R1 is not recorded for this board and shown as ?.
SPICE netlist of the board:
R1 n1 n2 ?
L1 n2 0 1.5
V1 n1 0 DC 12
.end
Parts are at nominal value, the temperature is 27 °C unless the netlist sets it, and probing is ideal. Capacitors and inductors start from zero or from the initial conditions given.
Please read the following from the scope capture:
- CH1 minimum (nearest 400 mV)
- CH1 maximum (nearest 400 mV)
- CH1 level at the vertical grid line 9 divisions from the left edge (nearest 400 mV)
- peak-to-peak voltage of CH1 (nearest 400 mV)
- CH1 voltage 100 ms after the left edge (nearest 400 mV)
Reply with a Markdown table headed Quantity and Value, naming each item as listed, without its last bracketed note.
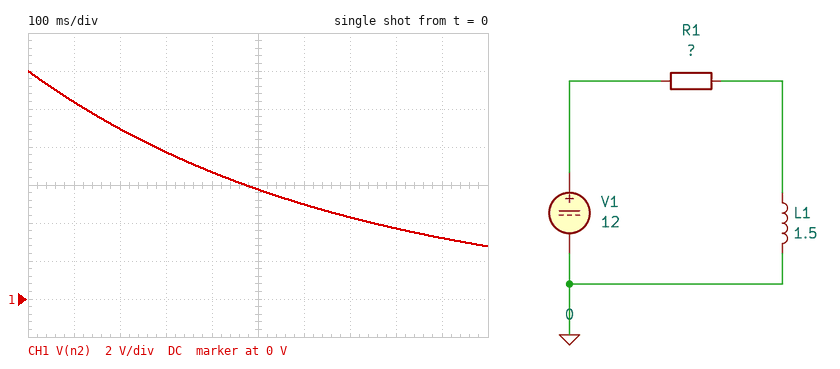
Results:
| Quantity | Value |
|---|---|
| CH1 minimum | 2.8 V |
| CH1 maximum | 12.0 V |
| CH1 level at the vertical grid line 9 divisions from the left edge | 3.2 V |
| peak-to-peak voltage of CH1 | 9.2 V |
| CH1 voltage 100 ms after the left edge | 10.4 V |
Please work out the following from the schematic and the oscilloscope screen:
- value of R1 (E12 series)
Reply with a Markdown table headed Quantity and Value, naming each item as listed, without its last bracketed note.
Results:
| Quantity | Value |
|---|---|
| value of R1 | 2.2 Ω |
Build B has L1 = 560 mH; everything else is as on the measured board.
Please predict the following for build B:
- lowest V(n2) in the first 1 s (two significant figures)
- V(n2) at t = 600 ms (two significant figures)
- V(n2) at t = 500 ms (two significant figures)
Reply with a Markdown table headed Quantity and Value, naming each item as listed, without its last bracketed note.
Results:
| Quantity | Value |
|---|---|
| lowest V(n2) in the first 1 s | 240 mV |
| V(n2) at t = 600 ms | 1.1 V |
| V(n2) at t = 500 ms | 1.7 V |
